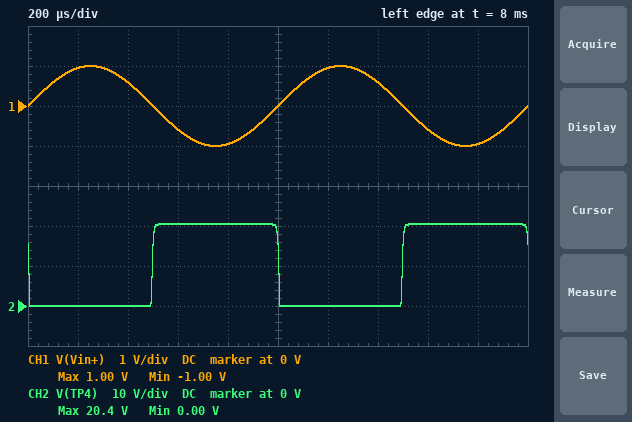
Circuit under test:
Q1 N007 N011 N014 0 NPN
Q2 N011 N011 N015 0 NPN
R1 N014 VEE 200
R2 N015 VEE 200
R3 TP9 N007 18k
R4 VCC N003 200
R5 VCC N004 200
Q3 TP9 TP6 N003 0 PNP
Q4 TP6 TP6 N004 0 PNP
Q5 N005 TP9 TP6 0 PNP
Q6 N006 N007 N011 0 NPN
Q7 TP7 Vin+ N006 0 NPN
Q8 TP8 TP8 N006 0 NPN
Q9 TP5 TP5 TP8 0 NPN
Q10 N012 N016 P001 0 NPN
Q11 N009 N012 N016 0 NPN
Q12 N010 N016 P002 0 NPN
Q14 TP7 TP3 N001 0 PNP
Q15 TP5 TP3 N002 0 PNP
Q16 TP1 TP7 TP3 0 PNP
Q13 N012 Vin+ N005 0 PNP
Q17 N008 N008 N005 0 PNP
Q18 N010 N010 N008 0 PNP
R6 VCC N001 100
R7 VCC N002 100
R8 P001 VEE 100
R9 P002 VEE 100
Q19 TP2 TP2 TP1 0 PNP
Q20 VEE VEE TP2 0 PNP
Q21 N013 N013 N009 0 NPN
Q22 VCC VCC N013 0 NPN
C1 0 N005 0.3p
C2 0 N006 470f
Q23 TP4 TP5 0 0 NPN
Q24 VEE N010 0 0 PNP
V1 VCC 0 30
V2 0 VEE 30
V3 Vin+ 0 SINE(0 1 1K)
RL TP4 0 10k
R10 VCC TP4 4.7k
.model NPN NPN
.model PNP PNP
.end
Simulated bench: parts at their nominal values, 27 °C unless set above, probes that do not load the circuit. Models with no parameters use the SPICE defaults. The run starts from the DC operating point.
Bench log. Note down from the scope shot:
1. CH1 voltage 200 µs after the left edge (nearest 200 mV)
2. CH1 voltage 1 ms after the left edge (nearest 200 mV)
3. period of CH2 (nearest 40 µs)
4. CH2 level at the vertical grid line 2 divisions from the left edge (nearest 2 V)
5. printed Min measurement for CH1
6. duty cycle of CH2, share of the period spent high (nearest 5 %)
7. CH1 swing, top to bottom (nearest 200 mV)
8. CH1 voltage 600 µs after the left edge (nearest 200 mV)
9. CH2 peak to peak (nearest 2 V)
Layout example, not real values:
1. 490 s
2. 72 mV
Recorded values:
1. 1.0 V
2. 0 V
3. 1.00 ms
4. 0 V
5. -1.00 V
6. 50 %
7. 2.0 V
8. -600 mV
9. 20 V
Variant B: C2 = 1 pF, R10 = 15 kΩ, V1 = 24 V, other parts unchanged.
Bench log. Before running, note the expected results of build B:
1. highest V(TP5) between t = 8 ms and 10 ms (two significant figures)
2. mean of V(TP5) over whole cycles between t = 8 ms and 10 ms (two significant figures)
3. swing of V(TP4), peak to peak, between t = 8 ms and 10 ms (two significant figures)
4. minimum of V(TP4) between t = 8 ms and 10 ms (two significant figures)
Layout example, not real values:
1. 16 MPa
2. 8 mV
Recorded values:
1. 820 mV
2. 480 mV
3. 9.6 V
4. 25 mV
